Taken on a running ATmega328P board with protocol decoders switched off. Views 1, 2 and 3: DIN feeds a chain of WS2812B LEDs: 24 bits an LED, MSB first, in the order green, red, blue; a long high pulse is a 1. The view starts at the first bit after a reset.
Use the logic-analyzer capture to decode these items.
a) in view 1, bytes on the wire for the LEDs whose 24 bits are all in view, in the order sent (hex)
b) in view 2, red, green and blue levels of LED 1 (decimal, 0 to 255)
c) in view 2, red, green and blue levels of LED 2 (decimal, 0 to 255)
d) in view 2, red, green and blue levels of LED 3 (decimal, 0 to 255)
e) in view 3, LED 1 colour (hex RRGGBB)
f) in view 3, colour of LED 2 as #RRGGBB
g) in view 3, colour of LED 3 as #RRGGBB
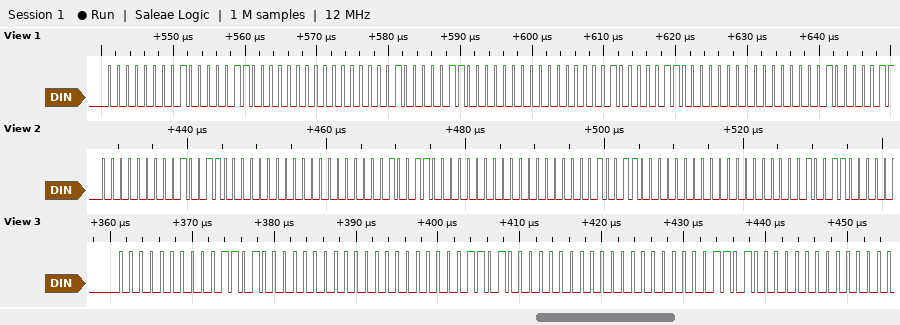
00 83 00 00 83 00 00 83 00
76, 0, 0
76, 0, 0
76, 0, 0
#340000
#340000
#340000
